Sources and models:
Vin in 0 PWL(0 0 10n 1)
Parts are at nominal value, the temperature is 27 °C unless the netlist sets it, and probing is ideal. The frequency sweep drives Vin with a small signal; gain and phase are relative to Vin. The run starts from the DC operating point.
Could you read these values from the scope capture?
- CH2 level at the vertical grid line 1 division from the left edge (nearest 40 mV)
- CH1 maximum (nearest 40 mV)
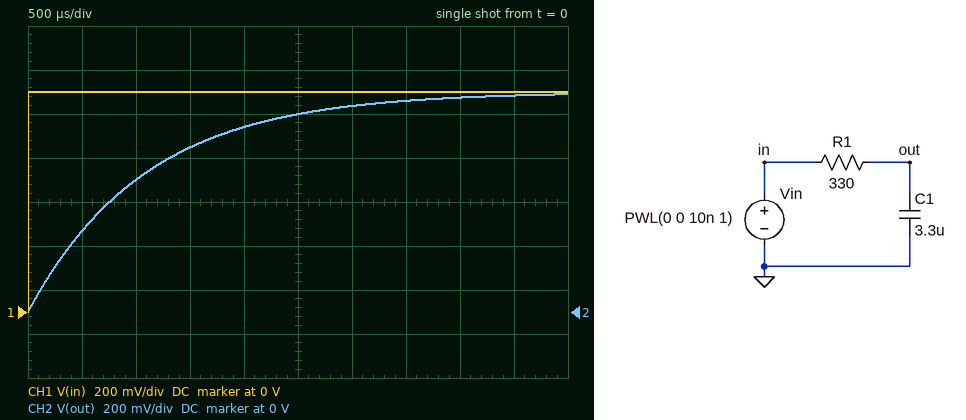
360 mV
1.00 V
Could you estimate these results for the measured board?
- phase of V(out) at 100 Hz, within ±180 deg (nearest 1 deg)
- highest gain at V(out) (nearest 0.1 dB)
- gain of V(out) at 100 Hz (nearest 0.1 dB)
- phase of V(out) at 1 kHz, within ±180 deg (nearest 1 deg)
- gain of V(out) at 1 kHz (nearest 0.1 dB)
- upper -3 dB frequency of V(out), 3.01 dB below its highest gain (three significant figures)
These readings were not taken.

-34 deg
0 dB
-1.7 dB
-82 deg
-16.8 dB
146 Hz
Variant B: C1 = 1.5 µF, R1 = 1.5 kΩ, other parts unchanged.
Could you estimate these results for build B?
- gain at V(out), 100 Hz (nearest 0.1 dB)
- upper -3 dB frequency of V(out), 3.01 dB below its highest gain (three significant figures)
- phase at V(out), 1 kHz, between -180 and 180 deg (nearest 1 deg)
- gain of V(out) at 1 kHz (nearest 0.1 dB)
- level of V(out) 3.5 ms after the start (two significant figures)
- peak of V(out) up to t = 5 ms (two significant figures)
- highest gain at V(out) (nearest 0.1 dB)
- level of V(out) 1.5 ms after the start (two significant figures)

-4.8 dB
70.7 Hz
-86 deg
-23.0 dB
790 mV
890 mV
0 dB
490 mV
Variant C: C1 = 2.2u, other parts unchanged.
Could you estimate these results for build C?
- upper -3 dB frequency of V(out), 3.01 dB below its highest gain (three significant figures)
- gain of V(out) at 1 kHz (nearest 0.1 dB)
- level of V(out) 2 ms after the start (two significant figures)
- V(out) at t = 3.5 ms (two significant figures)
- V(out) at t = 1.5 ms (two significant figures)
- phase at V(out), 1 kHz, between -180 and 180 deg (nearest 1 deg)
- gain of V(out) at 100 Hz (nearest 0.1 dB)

219 Hz
-13.4 dB
940 mV
990 mV
870 mV
-78 deg
-0.8 dB
